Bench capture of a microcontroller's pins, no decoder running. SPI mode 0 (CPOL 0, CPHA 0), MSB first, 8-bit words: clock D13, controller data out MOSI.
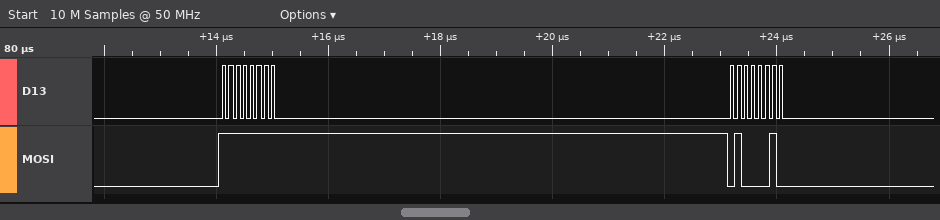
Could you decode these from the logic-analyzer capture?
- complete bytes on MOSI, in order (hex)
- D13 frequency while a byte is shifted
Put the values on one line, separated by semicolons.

FF 42; 8 MHz
